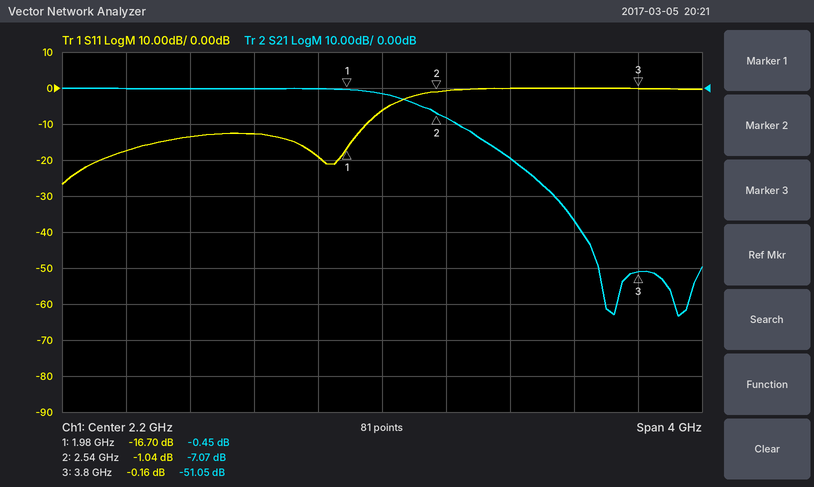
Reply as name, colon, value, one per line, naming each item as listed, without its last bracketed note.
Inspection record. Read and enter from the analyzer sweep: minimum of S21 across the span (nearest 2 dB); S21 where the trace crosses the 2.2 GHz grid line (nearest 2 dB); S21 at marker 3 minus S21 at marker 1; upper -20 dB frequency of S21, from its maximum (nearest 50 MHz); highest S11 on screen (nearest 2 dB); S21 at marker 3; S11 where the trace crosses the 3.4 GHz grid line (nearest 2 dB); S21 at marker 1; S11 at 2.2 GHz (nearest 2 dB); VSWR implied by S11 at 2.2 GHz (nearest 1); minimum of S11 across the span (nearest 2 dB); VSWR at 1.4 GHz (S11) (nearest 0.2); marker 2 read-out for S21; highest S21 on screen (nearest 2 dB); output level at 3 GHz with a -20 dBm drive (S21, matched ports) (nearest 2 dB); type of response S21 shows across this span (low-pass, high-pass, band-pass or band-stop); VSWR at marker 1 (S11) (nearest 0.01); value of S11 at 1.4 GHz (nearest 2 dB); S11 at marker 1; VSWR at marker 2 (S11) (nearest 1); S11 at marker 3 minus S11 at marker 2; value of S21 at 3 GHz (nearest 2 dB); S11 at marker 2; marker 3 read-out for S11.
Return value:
minimum of S21 across the span: -64 dB
S21 where the trace crosses the 2.2 GHz grid line: -2 dB
S21 at marker 3 minus S21 at marker 1: -50.60 dB
upper -20 dB frequency of S21, from its maximum: 3.00 GHz
highest S11 on screen: 0 dB
S21 at marker 3: -51.05 dB
S11 where the trace crosses the 3.4 GHz grid line: 0 dB
S21 at marker 1: -0.45 dB
S11 at 2.2 GHz: -6 dB
VSWR implied by S11 at 2.2 GHz: 3
minimum of S11 across the span: -26 dB
VSWR at 1.4 GHz (S11): 1.6
marker 2 read-out for S21: -7.07 dB
highest S21 on screen: 0 dB
output level at 3 GHz with a -20 dBm drive (S21, matched ports): -40 dBm
type of response S21 shows across this span: low-pass
VSWR at marker 1 (S11): 1.34
value of S11 at 1.4 GHz: -12 dB
S11 at marker 1: -16.70 dB
VSWR at marker 2 (S11): 17
S11 at marker 3 minus S11 at marker 2: 0.88 dB
value of S21 at 3 GHz: -20 dB
S11 at marker 2: -1.04 dB
marker 3 read-out for S11: -0.16 dB
